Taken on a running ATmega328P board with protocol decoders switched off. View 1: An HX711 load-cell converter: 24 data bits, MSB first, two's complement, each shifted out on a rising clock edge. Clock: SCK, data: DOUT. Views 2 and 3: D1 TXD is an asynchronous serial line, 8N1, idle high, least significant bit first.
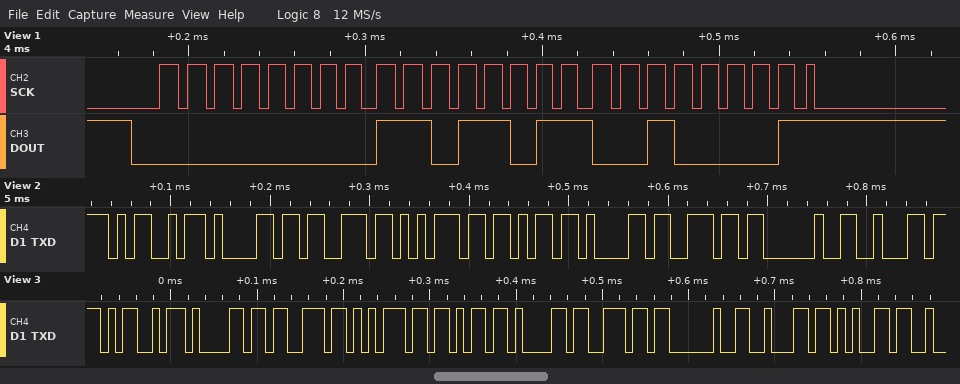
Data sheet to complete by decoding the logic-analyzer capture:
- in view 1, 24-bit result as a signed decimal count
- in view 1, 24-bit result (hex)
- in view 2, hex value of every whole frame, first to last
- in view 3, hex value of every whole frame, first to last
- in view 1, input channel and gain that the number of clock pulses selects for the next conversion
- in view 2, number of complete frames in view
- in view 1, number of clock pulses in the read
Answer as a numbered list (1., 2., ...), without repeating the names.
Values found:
1. 56097
2. 0x00DB21
3. 0x4D 0x61 0x73 0x75 0x6B 0x61 0x6E 0x20 0x62
4. 4D 61 73 75 6B 61 6E 20 62 65
5. channel A, gain 128
6. 9
7. 25
